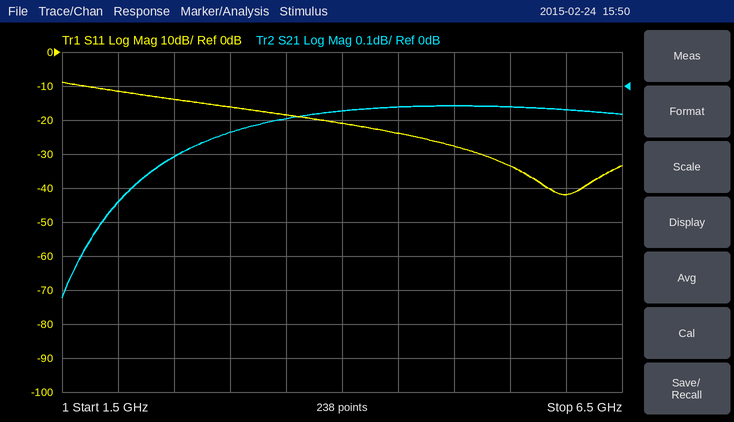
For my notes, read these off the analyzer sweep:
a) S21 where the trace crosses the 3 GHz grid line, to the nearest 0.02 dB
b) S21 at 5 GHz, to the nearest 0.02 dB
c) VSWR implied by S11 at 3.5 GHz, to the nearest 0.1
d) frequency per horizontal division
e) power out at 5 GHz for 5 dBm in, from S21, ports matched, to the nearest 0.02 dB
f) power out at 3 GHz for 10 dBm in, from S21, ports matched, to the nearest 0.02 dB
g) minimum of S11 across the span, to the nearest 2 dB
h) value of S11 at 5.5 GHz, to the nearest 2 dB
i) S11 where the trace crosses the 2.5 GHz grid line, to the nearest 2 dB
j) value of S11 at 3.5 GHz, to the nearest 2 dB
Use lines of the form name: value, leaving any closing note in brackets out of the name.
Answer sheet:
S21 where the trace crosses the 3 GHz grid line, to the nearest 0.02 dB: -0.14 dB
S21 at 5 GHz, to the nearest 0.02 dB: -0.06 dB
VSWR implied by S11 at 3.5 GHz, to the nearest 0.1: 1.3
frequency per horizontal division: 500 MHz
power out at 5 GHz for 5 dBm in, from S21, ports matched, to the nearest 0.02 dB: 4.94 dBm
power out at 3 GHz for 10 dBm in, from S21, ports matched, to the nearest 0.02 dB: 9.86 dBm
minimum of S11 across the span, to the nearest 2 dB: -42 dB
value of S11 at 5.5 GHz, to the nearest 2 dB: -34 dB
S11 where the trace crosses the 2.5 GHz grid line, to the nearest 2 dB: -14 dB
value of S11 at 3.5 GHz, to the nearest 2 dB: -18 dB
